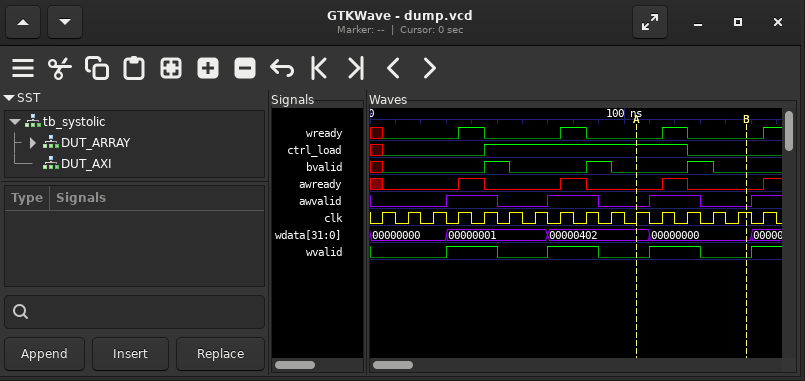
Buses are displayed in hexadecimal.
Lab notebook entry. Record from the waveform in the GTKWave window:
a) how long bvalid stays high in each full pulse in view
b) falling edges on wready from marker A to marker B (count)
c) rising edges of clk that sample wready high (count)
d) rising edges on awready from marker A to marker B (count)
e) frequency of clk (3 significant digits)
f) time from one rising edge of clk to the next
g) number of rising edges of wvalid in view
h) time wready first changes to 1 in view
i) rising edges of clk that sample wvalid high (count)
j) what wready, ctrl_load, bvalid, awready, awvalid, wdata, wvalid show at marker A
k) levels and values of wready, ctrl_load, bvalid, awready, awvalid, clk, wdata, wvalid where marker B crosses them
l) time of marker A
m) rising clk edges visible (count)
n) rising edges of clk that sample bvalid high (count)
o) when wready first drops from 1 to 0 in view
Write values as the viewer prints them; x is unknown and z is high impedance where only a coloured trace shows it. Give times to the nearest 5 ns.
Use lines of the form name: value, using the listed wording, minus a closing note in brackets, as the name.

how long bvalid stays high in each full pulse in view: 10 ns, 10 ns, 10 ns
falling edges on wready from marker A to marker B: 1
rising edges of clk that sample wready high: 3
rising edges on awready from marker A to marker B: 1
frequency of clk: 100 MHz
time from one rising edge of clk to the next: 10 ns
number of rising edges of wvalid in view: 4
time wready first changes to 1 in view: 35 ns
rising edges of clk that sample wvalid high: 7
what wready, ctrl_load, bvalid, awready, awvalid, wdata, wvalid show at marker A: wready=0, ctrl_load=1, bvalid=0, awready=0, awvalid=0, wdata=00000402, wvalid=0
levels and values of wready, ctrl_load, bvalid, awready, awvalid, clk, wdata, wvalid where marker B crosses them: wready=0, ctrl_load=0, bvalid=0, awready=0, awvalid=0, clk=1, wdata=00000000, wvalid=0
time of marker A: 105 ns
rising clk edges visible: 16
rising edges of clk that sample bvalid high: 3
when wready first drops from 1 to 0 in view: 45 ns
